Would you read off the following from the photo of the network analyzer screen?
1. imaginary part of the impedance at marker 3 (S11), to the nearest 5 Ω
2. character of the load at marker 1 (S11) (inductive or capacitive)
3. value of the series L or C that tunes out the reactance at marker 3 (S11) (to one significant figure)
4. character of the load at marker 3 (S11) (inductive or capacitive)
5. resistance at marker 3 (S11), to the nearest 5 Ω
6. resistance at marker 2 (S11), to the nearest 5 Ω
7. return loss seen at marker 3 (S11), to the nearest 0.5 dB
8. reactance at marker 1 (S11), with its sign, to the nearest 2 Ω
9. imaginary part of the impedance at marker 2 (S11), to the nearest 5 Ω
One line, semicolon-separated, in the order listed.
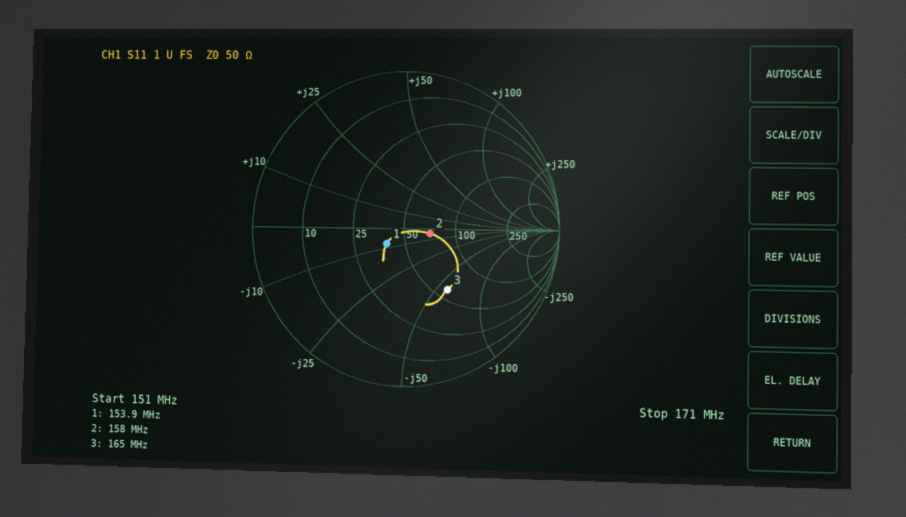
-60 Ω; capacitive; 60 nH; capacitive; 60 Ω; 70 Ω; 6.5 dB; -8 Ω; -5 Ω
